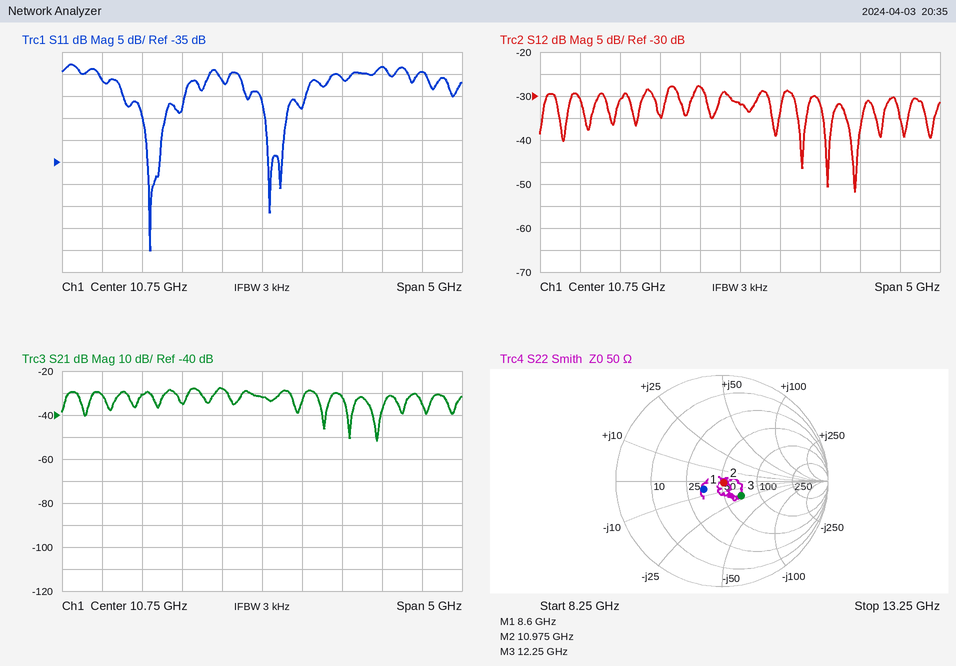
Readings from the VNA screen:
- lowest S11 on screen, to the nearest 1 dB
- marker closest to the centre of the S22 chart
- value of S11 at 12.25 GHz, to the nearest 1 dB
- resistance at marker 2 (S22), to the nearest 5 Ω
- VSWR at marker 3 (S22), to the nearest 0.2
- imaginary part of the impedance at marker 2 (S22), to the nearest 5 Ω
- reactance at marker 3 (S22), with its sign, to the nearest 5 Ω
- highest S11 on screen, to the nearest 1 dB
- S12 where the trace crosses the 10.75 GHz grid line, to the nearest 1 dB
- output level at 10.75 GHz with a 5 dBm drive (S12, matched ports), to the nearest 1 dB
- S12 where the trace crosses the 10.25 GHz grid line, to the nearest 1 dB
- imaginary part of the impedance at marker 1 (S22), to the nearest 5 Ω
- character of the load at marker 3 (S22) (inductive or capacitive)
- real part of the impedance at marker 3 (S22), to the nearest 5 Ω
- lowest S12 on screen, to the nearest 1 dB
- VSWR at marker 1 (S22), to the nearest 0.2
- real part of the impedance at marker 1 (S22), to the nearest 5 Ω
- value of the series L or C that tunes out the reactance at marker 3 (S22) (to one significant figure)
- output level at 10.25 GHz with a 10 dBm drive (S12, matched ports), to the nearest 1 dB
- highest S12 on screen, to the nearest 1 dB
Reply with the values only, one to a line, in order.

-55 dB
marker 2
-13 dB
50 Ω
1.6
0 Ω
-20 Ω
-13 dB
-32 dB
-27 dBm
-28 dB
-5 Ω
capacitive
70 Ω
-52 dB
1.4
35 Ω
300 pH
-18 dBm
-28 dB
